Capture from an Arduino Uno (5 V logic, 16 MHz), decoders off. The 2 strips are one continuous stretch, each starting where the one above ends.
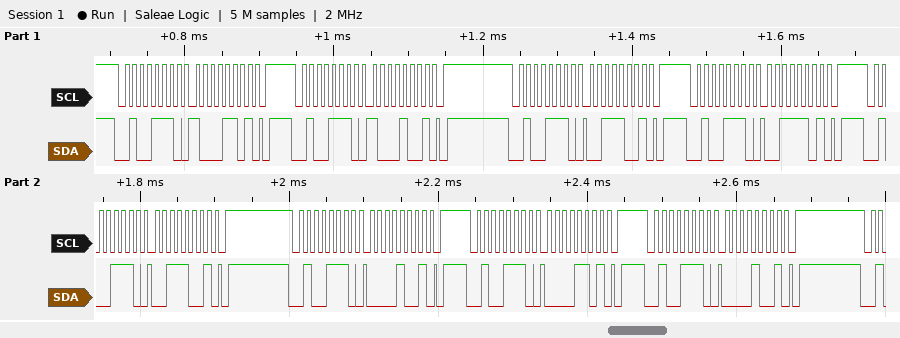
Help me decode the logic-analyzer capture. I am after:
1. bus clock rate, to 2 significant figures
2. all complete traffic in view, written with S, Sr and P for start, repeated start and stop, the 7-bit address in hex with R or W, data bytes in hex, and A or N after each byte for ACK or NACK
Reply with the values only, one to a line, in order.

100 kHz
S 27W A 8D A P S 27W A 89 A P S 27W A 39 A P S 27W A 3D A P S 27W A 39 A P S 27W A 09 A P S 27W A 0D A P S 27W A 09 A P
